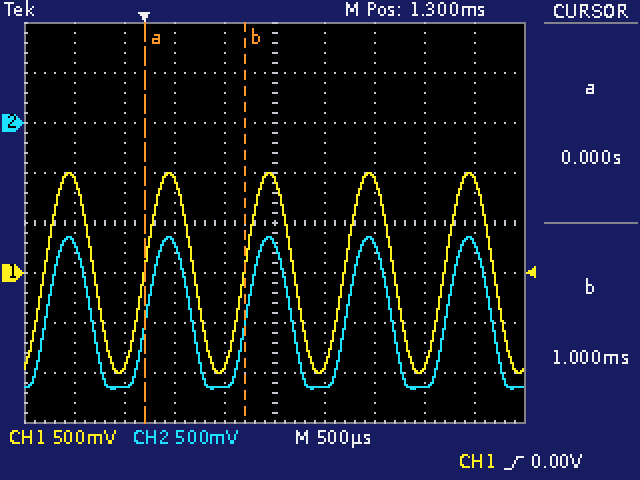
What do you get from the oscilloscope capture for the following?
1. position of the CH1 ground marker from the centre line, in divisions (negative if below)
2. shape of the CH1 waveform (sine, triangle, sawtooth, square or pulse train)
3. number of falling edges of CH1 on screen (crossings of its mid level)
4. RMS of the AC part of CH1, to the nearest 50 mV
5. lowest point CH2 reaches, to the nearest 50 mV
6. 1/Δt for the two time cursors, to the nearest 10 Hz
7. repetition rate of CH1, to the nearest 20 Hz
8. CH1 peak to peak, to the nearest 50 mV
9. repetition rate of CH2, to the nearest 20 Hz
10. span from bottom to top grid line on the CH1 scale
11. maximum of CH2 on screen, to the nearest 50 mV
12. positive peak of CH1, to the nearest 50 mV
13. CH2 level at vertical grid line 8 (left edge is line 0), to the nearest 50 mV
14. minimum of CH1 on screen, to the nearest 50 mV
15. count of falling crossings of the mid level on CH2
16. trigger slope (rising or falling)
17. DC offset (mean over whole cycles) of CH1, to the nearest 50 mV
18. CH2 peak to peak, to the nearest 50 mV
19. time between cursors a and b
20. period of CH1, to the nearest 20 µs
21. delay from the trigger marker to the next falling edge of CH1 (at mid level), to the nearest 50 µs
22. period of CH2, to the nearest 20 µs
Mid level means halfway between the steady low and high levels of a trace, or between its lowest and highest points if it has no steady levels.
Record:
-1.0 div
sine
5
700 mV
-2.65 V
1.00 kHz
1.00 kHz
2.00 V
1.00 kHz
4 V
-1.15 V
1.00 V
-2.65 V
-1.00 V
5
rising
0 mV
1.50 V
1.00 ms
1.00 ms
500 µs
1.00 ms
